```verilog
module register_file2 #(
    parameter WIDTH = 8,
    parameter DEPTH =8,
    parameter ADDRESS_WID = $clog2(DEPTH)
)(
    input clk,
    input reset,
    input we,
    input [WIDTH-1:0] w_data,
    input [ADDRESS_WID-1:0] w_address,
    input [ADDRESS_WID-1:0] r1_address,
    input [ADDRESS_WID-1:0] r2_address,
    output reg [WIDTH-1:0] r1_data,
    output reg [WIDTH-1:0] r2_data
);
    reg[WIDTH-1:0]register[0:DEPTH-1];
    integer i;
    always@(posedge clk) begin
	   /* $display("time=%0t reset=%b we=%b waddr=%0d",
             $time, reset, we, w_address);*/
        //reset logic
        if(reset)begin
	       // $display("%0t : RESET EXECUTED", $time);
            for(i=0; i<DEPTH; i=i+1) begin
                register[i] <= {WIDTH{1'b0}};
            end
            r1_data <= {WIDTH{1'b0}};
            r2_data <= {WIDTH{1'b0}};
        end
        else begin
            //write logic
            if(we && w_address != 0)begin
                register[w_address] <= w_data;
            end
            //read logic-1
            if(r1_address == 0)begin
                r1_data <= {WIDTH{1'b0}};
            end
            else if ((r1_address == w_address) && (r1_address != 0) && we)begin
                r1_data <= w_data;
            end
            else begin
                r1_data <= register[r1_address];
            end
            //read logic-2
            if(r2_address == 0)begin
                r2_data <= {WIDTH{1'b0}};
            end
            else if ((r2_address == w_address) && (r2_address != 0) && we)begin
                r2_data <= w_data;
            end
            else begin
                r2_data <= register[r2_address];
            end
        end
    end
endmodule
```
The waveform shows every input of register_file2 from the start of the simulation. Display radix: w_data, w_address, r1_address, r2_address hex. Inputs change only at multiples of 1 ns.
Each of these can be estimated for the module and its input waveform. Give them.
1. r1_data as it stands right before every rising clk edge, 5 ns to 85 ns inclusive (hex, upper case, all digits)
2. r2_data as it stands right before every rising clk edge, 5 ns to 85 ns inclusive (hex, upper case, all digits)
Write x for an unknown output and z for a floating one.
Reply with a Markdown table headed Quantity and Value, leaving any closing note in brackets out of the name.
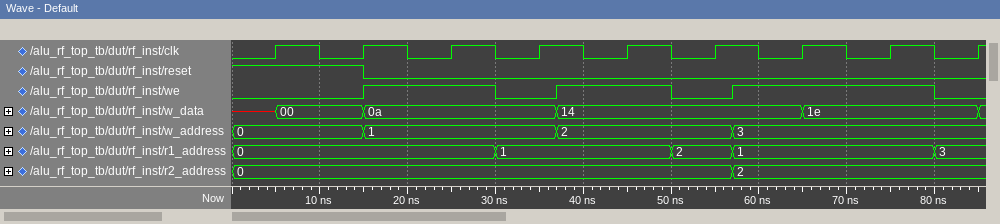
| Quantity | Value |
|---|---|
| r1_data as it stands right before every rising clk edge, 5 ns to 85 ns inclusive | x, 00, 00, 00, 0A, 0A, 14, 0A, 0A |
| r2_data as it stands right before every rising clk edge, 5 ns to 85 ns inclusive | x, 00, 00, 00, 00, 00, 00, 14, 14 |
